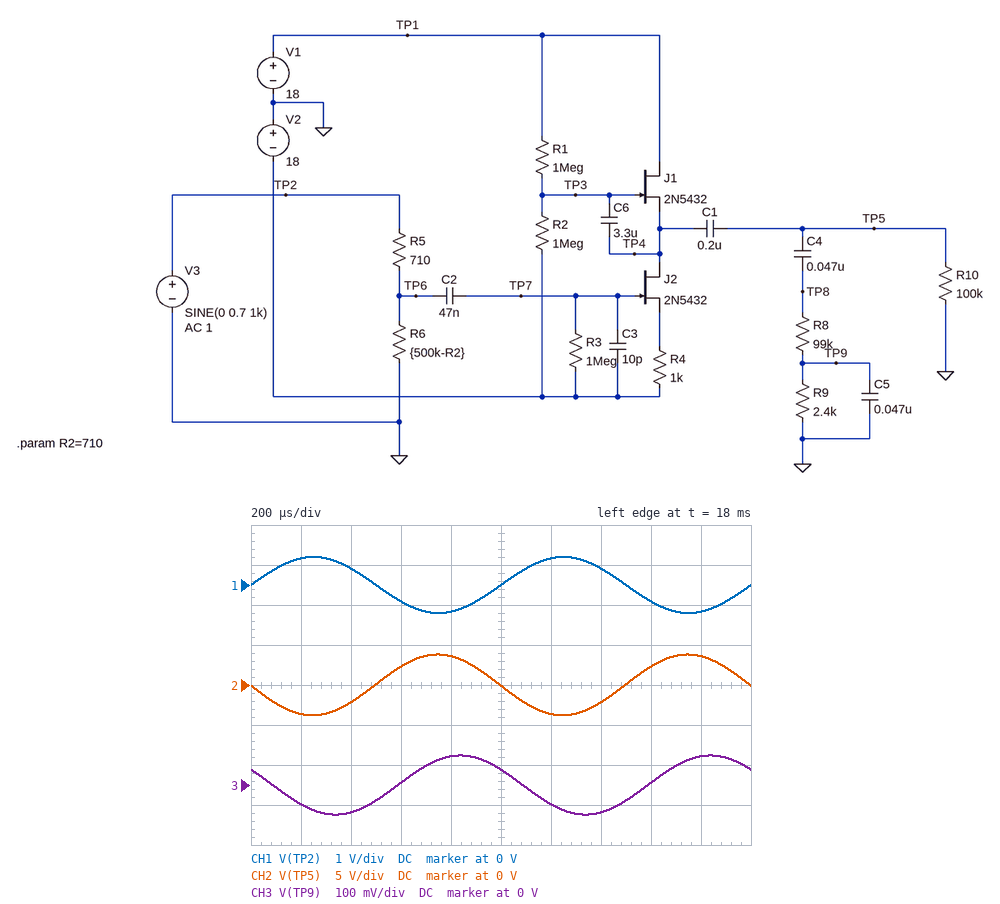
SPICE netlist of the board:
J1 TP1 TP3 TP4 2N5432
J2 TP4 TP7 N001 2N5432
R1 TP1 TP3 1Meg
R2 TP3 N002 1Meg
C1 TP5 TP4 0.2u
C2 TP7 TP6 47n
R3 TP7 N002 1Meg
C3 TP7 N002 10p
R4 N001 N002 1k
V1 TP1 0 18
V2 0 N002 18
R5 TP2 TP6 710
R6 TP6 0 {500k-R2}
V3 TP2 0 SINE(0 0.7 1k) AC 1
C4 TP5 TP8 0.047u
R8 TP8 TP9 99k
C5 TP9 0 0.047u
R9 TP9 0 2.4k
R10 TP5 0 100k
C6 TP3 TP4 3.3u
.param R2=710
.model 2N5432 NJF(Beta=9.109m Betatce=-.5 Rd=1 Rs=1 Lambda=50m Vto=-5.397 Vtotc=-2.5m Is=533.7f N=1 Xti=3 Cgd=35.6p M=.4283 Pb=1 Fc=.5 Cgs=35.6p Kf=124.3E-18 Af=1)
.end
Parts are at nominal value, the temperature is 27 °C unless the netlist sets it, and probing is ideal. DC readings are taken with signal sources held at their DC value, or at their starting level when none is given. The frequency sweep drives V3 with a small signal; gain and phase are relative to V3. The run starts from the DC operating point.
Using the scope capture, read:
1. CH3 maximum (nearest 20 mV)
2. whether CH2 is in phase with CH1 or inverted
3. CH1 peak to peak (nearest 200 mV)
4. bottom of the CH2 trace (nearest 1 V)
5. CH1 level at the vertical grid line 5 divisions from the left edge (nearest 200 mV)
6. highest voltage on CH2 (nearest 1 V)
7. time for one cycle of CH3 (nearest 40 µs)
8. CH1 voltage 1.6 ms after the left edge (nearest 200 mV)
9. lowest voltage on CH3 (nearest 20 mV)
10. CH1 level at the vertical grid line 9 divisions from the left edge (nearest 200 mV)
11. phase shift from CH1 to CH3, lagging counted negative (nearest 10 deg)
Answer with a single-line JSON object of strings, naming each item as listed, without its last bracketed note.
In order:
{"CH3 maximum": "80 mV", "whether CH2 is in phase with CH1 or inverted": "inverted", "CH1 peak to peak": "1.4 V", "bottom of the CH2 trace": "-4 V", "CH1 level at the vertical grid line 5 divisions from the left edge": "0 V", "highest voltage on CH2": "4 V", "time for one cycle of CH3": "1.00 ms", "CH1 voltage 1.6 ms after the left edge": "-400 mV", "lowest voltage on CH3": "-80 mV", "CH1 level at the vertical grid line 9 divisions from the left edge": "-600 mV", "phase shift from CH1 to CH3, lagging counted negative": "150 deg"}
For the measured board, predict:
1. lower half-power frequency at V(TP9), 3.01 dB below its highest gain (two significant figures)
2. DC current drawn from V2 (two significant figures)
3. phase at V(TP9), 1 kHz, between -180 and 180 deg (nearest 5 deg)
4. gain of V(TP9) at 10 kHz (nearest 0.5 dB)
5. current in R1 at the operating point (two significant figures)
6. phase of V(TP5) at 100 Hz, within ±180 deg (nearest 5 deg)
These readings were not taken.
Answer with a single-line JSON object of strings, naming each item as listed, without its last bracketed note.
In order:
{"lower half-power frequency at V(TP9), 3.01 dB below its highest gain": "40 Hz", "DC current drawn from V2": "4.9 mA", "phase at V(TP9), 1 kHz, between -180 and 180 deg": "150 deg", "gain of V(TP9) at 10 kHz": "-34.5 dB", "current in R1 at the operating point": "18 µA", "phase of V(TP5) at 100 Hz, within ±180 deg": "-165 deg"}
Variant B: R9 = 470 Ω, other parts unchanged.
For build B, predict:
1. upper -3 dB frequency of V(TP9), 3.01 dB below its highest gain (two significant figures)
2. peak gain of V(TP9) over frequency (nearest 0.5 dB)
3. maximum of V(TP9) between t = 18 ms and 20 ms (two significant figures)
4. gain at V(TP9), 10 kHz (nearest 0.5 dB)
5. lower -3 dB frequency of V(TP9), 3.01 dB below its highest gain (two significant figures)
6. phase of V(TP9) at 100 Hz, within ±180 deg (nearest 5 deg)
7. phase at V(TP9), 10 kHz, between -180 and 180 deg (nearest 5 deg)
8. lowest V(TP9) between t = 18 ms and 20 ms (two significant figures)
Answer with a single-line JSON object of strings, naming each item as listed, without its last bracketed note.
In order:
{"upper -3 dB frequency of V(TP9), 3.01 dB below its highest gain": "7.3 kHz", "peak gain of V(TP9) over frequency": "-32.0 dB", "maximum of V(TP9) between t = 18 ms and 20 ms": "18 mV", "gain at V(TP9), 10 kHz": "-36.5 dB", "lower -3 dB frequency of V(TP9), 3.01 dB below its highest gain": "42 Hz", "phase of V(TP9) at 100 Hz, within ±180 deg": "-150 deg", "phase at V(TP9), 10 kHz, between -180 and 180 deg": "125 deg", "lowest V(TP9) between t = 18 ms and 20 ms": "-18 mV"}
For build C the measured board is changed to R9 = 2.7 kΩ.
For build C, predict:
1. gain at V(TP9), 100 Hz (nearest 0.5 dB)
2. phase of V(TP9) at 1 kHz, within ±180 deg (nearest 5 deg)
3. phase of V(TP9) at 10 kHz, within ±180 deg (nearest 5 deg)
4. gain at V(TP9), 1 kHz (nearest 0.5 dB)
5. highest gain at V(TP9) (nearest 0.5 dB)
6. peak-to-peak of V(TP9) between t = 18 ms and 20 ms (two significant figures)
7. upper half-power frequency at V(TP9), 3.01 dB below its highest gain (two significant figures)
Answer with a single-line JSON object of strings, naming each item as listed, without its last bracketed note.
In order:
{"gain at V(TP9), 100 Hz": "-17.5 dB", "phase of V(TP9) at 1 kHz, within ±180 deg": "145 deg", "phase of V(TP9) at 10 kHz, within ±180 deg": "95 deg", "gain at V(TP9), 1 kHz": "-19.0 dB", "highest gain at V(TP9)": "-17.0 dB", "peak-to-peak of V(TP9) between t = 18 ms and 20 ms": "160 mV", "upper half-power frequency at V(TP9), 3.01 dB below its highest gain": "1.4 kHz"}
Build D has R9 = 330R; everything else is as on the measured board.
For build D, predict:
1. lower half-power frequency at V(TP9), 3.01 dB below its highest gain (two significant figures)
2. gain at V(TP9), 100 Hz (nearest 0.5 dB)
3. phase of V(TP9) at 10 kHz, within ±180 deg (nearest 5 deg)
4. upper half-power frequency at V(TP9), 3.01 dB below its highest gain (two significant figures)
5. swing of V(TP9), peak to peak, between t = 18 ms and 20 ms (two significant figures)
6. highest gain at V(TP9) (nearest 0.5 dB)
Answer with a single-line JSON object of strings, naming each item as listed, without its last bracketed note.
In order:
{"lower half-power frequency at V(TP9), 3.01 dB below its highest gain": "42 Hz", "gain at V(TP9), 100 Hz": "-35.5 dB", "phase of V(TP9) at 10 kHz, within ±180 deg": "135 deg", "upper half-power frequency at V(TP9), 3.01 dB below its highest gain": "10 kHz", "swing of V(TP9), peak to peak, between t = 18 ms and 20 ms": "25 mV", "highest gain at V(TP9)": "-35.0 dB"}
